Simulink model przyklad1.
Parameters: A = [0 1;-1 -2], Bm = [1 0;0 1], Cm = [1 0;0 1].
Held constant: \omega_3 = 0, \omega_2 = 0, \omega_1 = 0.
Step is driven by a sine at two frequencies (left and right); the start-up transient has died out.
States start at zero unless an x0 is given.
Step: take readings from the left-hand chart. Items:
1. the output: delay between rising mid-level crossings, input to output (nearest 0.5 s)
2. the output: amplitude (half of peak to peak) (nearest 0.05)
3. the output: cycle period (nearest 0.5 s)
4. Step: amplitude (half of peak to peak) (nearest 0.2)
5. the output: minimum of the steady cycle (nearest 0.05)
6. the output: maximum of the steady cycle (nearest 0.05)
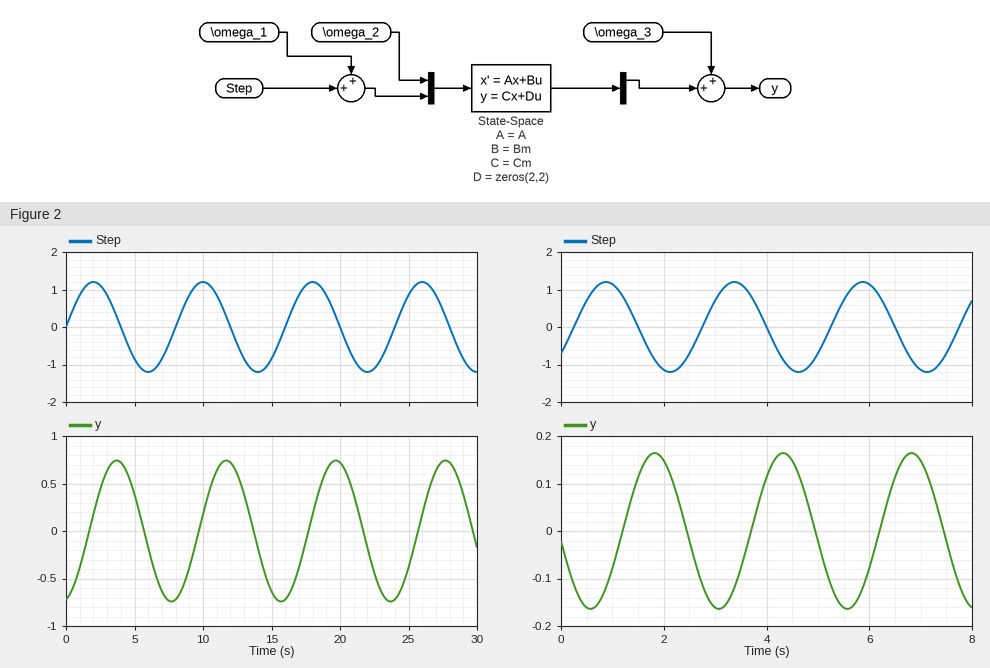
1.5 s
0.75
8.0 s
1.2
-0.75
0.75
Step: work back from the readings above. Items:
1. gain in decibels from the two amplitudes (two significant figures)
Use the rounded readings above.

-4.1 dB
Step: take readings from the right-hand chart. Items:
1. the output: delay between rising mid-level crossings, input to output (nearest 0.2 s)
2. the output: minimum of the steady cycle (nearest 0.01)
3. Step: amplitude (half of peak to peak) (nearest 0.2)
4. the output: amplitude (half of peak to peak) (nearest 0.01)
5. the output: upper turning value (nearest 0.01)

1.0 s
-0.16
1.2
0.16
0.16
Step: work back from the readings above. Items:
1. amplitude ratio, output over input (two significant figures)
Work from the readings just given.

0.13
